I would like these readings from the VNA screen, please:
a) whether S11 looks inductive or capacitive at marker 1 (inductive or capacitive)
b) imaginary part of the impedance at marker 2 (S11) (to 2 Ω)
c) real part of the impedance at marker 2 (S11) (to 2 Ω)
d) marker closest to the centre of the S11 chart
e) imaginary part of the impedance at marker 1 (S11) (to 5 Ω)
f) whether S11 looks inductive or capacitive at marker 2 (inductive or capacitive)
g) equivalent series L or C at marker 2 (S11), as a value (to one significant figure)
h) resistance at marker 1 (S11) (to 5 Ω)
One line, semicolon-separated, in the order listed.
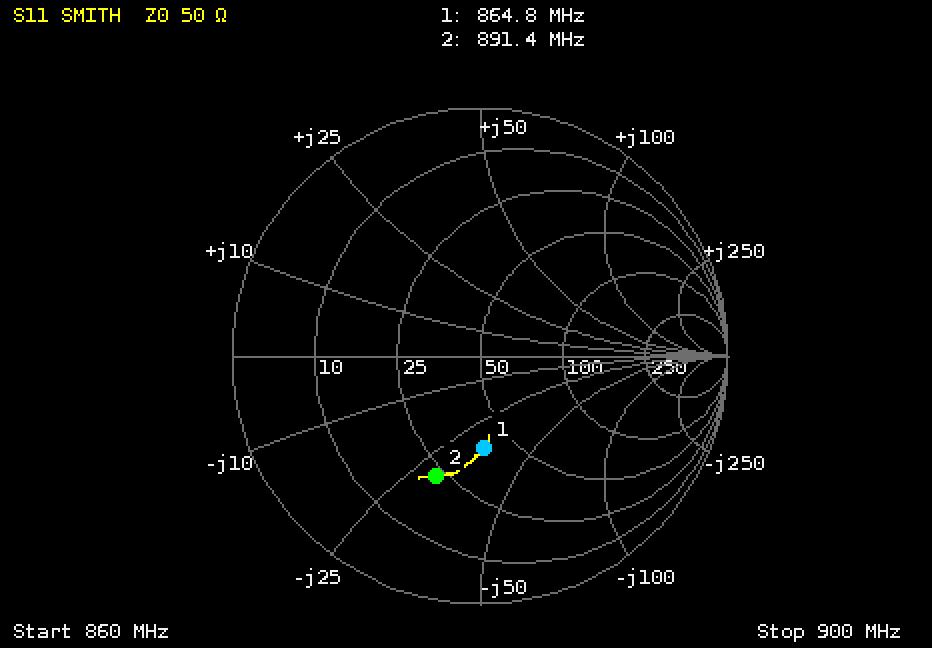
capacitive; -30 Ω; 22 Ω; marker 1; -35 Ω; capacitive; 6 pF; 40 Ω
